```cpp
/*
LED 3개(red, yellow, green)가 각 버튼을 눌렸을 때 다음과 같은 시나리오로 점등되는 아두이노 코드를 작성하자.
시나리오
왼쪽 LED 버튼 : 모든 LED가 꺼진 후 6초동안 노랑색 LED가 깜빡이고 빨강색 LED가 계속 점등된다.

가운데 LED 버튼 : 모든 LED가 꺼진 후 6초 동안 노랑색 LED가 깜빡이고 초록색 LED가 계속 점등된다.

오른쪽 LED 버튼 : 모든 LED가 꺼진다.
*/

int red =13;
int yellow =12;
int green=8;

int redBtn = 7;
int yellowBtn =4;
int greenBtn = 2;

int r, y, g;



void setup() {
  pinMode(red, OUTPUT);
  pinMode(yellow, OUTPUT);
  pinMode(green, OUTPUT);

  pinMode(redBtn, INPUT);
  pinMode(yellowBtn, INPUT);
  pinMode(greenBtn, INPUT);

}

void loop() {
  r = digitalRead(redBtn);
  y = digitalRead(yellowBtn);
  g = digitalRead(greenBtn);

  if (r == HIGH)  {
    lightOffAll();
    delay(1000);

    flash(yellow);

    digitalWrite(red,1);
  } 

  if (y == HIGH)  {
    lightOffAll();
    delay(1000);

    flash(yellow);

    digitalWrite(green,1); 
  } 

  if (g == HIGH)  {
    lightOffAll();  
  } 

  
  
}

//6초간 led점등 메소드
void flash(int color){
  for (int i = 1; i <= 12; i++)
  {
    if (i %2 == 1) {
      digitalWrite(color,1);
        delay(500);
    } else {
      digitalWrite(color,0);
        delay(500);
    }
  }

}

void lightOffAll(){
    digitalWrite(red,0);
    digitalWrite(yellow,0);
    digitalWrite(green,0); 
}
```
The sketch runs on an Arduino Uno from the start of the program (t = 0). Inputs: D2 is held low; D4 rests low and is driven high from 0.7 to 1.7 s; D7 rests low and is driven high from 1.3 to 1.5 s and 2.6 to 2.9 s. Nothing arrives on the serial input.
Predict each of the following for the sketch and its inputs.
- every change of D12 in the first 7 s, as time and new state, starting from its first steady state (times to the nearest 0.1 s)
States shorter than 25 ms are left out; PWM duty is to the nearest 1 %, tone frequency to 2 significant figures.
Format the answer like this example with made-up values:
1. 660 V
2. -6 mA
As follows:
1. 0 s low; 1.7 s high; 2.2 s low; 2.7 s high; 3.2 s low; 3.7 s high; 4.2 s low; 4.7 s high; 5.2 s low; 5.7 s high; 6.2 s low; 6.7 s high
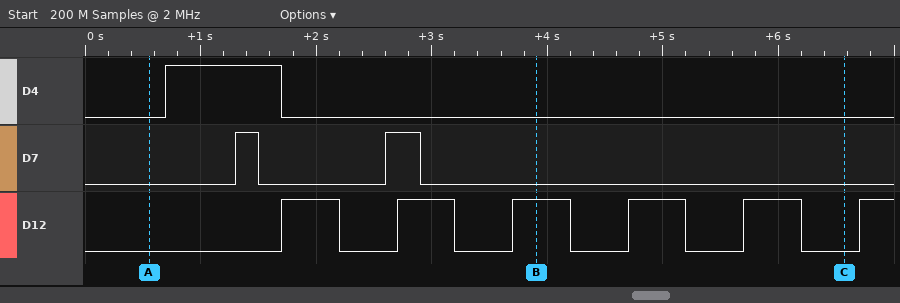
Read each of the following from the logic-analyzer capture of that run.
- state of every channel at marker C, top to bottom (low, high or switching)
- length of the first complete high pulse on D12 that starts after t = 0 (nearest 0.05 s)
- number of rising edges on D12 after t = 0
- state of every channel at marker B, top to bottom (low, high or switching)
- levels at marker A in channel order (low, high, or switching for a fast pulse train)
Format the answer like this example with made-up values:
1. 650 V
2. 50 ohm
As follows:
1. D4 low, D7 low, D12 low
2. 0.50 s
3. 6
4. D4 low, D7 low, D12 high
5. D4 low, D7 low, D12 low
